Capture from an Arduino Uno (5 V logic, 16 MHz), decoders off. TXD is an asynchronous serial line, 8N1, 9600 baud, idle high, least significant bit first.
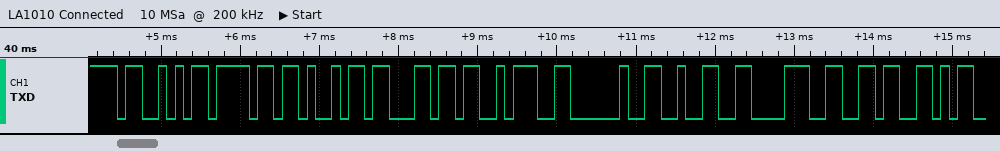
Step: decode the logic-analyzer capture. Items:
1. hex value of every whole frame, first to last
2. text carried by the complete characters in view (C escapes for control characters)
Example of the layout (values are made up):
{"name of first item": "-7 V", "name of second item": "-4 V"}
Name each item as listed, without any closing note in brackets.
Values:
{"hex value of every whole frame, first to last": "0x53 0x6F 0x69 0x6C 0x3A 0x20 0x32 0x38 0x36", "text carried by the complete characters in view": "\"Soil: 286\""}
